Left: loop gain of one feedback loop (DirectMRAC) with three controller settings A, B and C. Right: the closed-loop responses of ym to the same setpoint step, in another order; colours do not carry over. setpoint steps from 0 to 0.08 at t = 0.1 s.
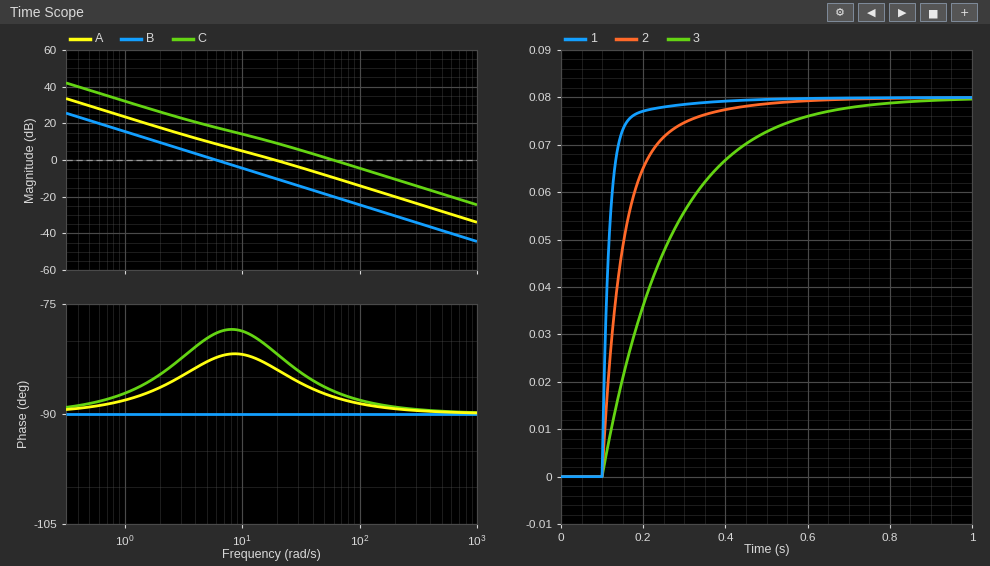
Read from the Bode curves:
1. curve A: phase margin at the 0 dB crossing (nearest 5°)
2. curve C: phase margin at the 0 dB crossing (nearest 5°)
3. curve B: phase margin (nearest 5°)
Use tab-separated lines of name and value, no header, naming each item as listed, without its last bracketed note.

curve A: phase margin at the 0 dB crossing	95°
curve C: phase margin at the 0 dB crossing	95°
curve B: phase margin	90°
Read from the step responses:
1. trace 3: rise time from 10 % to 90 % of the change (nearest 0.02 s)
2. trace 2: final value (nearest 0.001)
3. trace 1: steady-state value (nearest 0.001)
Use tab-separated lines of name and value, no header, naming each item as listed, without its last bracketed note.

trace 3: rise time from 10 % to 90 % of the change	0.36 s
trace 2: final value	0.080
trace 1: steady-state value	0.080
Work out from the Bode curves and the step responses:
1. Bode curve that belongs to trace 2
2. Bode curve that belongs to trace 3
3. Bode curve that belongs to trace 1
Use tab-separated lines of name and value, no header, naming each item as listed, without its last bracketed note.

Bode curve that belongs to trace 2	A
Bode curve that belongs to trace 3	B
Bode curve that belongs to trace 1	C
